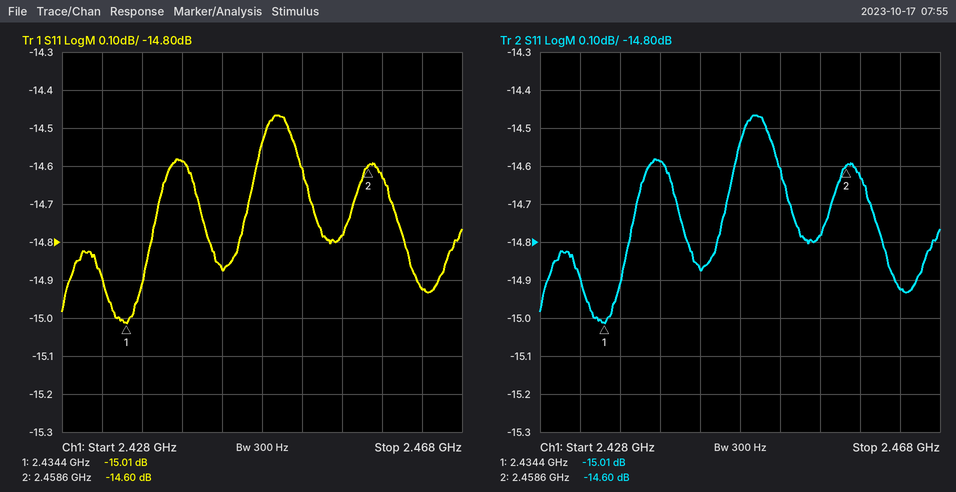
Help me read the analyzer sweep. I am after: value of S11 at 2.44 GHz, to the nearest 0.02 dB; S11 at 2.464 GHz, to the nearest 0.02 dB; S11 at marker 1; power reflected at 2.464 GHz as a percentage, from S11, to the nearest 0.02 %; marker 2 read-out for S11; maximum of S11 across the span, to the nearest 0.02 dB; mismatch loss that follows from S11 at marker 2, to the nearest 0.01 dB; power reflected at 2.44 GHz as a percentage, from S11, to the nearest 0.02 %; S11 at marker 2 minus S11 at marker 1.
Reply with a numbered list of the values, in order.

1. -14.58 dB
2. -14.92 dB
3. -15.01 dB
4. 3.22 %
5. -14.60 dB
6. -14.46 dB
7. 0.15 dB
8. 3.48 %
9. 0.41 dB
